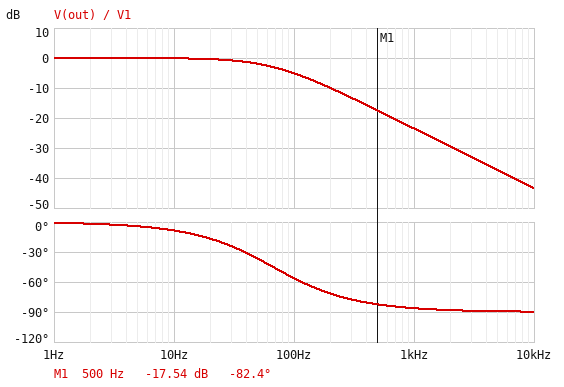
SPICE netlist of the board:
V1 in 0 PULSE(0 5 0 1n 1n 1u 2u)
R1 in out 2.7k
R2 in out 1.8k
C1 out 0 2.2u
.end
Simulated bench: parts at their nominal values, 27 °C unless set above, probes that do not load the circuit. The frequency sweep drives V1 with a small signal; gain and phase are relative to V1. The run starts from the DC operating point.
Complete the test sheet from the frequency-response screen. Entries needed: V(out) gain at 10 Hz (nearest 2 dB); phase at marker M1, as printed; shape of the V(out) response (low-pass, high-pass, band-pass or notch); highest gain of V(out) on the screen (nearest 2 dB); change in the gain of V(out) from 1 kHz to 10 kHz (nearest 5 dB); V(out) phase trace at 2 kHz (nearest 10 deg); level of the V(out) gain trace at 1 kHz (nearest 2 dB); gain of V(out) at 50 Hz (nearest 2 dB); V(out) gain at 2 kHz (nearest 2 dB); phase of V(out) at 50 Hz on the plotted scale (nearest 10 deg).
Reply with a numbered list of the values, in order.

1. 0 dB
2. -82.4 deg
3. low-pass
4. 0 dB
5. -20 dB
6. -90 deg
7. -24 dB
8. -2 dB
9. -30 dB
10. -40 deg
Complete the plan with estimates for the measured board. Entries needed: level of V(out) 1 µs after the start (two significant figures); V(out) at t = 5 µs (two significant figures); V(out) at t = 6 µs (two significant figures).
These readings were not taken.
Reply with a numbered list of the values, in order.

1. 2.1 mV
2. 6.3 mV
3. 6.3 mV
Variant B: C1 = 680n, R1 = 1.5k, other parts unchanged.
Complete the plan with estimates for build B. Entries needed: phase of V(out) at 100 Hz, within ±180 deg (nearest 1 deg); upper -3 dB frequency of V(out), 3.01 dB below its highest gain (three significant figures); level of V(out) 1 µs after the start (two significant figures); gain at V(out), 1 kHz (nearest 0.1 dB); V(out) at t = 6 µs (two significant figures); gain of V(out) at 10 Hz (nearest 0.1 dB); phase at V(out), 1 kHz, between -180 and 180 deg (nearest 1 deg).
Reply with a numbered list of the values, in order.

1. -19 deg
2. 286 Hz
3. 9.0 mV
4. -11.2 dB
5. 27 mV
6. 0 dB
7. -74 deg
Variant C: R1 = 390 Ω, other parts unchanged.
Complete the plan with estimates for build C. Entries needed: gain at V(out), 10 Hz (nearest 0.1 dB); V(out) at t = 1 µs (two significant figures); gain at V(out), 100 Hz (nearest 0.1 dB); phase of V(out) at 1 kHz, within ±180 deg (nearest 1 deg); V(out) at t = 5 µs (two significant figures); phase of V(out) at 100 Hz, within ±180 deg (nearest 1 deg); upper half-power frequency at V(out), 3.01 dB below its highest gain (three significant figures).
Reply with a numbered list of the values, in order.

1. 0 dB
2. 7.1 mV
3. -0.8 dB
4. -77 deg
5. 21 mV
6. -24 deg
7. 226 Hz
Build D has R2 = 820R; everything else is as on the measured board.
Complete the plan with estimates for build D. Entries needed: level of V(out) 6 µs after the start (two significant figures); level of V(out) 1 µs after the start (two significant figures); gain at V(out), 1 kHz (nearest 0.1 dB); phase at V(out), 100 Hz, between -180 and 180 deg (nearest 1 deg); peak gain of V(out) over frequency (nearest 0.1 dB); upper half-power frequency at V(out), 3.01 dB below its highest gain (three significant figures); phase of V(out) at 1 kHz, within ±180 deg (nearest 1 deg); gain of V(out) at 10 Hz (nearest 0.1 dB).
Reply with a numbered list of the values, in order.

1. 11 mV
2. 3.6 mV
3. -18.8 dB
4. -41 deg
5. 0 dB
6. 115 Hz
7. -83 deg
8. 0 dB
